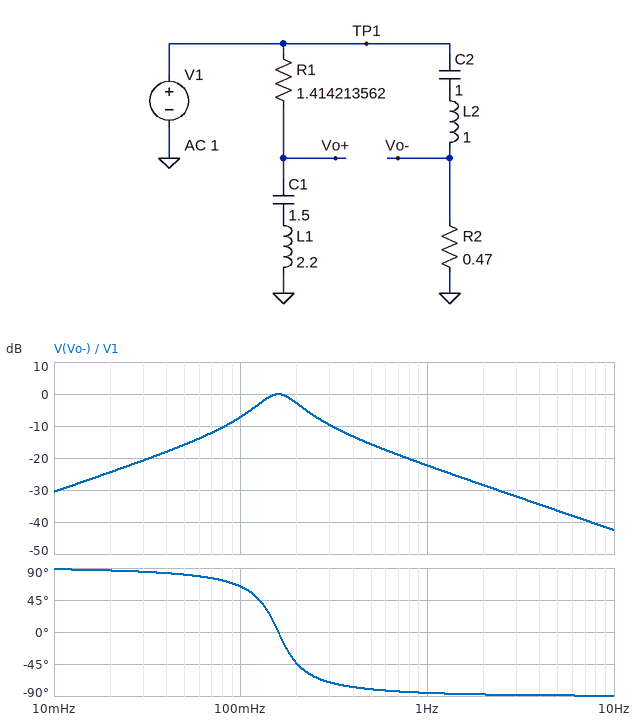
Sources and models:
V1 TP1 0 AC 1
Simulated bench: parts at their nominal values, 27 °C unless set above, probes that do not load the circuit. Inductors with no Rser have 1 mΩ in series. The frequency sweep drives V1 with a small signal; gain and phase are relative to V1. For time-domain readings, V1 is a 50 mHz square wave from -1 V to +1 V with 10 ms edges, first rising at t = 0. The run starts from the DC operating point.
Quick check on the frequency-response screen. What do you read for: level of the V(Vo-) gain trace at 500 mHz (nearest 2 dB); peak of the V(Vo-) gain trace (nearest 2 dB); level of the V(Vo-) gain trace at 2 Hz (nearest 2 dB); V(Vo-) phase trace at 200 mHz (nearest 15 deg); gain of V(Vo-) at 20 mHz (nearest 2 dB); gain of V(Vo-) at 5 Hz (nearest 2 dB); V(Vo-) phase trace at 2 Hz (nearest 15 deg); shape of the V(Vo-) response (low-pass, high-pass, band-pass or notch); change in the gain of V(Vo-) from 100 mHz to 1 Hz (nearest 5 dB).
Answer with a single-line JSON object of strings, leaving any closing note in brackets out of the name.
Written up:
{"level of the V(Vo-) gain trace at 500 mHz": "-16 dB", "peak of the V(Vo-) gain trace": "0 dB", "level of the V(Vo-) gain trace at 2 Hz": "-28 dB", "V(Vo-) phase trace at 200 mHz": "-45 deg", "gain of V(Vo-) at 20 mHz": "-24 dB", "gain of V(Vo-) at 5 Hz": "-36 dB", "V(Vo-) phase trace at 2 Hz": "-90 deg", "shape of the V(Vo-) response": "band-pass", "change in the gain of V(Vo-) from 100 mHz to 1 Hz": "-15 dB"}
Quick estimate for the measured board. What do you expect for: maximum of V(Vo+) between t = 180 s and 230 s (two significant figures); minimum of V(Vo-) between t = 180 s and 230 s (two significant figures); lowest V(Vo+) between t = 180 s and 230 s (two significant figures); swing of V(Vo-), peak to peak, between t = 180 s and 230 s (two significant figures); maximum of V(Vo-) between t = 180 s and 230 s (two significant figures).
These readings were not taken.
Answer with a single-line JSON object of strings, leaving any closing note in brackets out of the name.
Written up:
{"maximum of V(Vo+) between t = 180 s and 230 s": "1.1 V", "minimum of V(Vo-) between t = 180 s and 230 s": "-750 mV", "lowest V(Vo+) between t = 180 s and 230 s": "-1.1 V", "swing of V(Vo-), peak to peak, between t = 180 s and 230 s": "1.5 V", "maximum of V(Vo-) between t = 180 s and 230 s": "750 mV"}
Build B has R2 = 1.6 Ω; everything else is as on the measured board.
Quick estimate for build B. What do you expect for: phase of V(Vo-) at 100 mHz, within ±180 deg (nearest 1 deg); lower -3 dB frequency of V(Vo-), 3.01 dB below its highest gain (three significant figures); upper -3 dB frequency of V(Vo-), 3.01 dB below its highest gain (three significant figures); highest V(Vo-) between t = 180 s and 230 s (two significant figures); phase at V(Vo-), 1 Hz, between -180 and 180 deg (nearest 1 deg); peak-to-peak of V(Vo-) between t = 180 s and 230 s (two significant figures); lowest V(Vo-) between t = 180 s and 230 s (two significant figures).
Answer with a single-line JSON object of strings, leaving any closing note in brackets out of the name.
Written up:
{"phase of V(Vo-) at 100 mHz, within ±180 deg": "31 deg", "lower -3 dB frequency of V(Vo-), 3.01 dB below its highest gain": "76.5 mHz", "upper -3 dB frequency of V(Vo-), 3.01 dB below its highest gain": "331 mHz", "highest V(Vo-) between t = 180 s and 230 s": "1.4 V", "phase at V(Vo-), 1 Hz, between -180 and 180 deg": "-75 deg", "peak-to-peak of V(Vo-) between t = 180 s and 230 s": "2.7 V", "lowest V(Vo-) between t = 180 s and 230 s": "-1.4 V"}
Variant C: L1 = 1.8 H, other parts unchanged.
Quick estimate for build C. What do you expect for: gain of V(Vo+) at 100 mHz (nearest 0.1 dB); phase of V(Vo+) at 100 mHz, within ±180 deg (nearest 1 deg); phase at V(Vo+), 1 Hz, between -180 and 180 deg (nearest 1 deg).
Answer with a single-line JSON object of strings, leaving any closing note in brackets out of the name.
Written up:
{"gain of V(Vo+) at 100 mHz": "-26.1 dB", "phase of V(Vo+) at 100 mHz, within ±180 deg": "86 deg", "phase at V(Vo+), 1 Hz, between -180 and 180 deg": "7 deg"}
